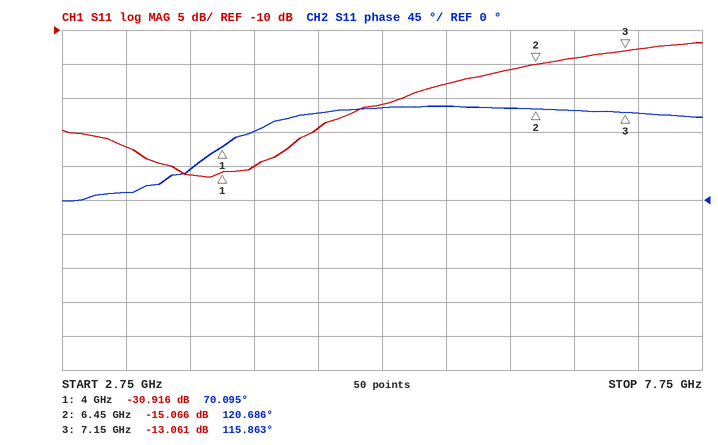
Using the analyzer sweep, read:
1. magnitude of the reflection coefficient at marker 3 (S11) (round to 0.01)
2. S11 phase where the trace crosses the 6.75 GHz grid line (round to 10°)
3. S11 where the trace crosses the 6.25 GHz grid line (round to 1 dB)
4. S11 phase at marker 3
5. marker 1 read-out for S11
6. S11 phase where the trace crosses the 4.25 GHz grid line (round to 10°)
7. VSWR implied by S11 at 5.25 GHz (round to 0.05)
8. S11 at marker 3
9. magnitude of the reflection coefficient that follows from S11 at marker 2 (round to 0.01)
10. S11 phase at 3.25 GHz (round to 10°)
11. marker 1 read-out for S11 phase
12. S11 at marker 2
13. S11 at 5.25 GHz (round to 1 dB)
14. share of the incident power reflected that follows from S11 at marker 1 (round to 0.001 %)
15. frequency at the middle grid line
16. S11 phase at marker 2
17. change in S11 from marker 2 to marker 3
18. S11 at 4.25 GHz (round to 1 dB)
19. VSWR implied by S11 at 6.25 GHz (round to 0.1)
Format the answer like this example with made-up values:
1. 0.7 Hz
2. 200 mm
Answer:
1. 0.22
2. 120°
3. -16 dB
4. 115.863°
5. -30.916 dB
6. 90°
7. 1.20
8. -13.061 dB
9. 0.18
10. 10°
11. 70.095°
12. -15.066 dB
13. -21 dB
14. 0.081 %
15. 5.25 GHz
16. 120.686°
17. 2.005 dB
18. -30 dB
19. 1.4
